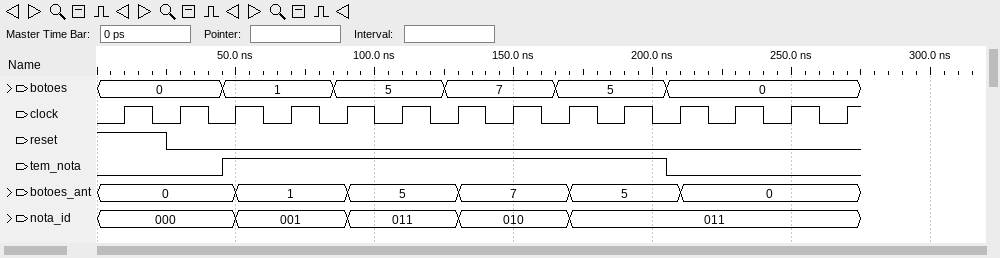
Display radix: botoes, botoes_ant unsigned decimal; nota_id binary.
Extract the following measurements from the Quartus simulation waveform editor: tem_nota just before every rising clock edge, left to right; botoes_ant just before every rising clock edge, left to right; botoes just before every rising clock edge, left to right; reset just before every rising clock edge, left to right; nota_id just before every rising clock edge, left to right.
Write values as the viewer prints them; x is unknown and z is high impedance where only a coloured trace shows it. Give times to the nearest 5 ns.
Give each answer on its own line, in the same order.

0 0 1 1 1 1 1 1 1 1 0 0 0 0
0, 0, 0, 1, 1, 5, 5, 7, 7, 5, 5, 0, 0, 0
0, 0, 1, 1, 5, 5, 7, 7, 5, 5, 0, 0, 0, 0
1 0 0 0 0 0 0 0 0 0 0 0 0 0
000, 000, 000, 001, 001, 011, 011, 010, 010, 011, 011, 011, 011, 011
